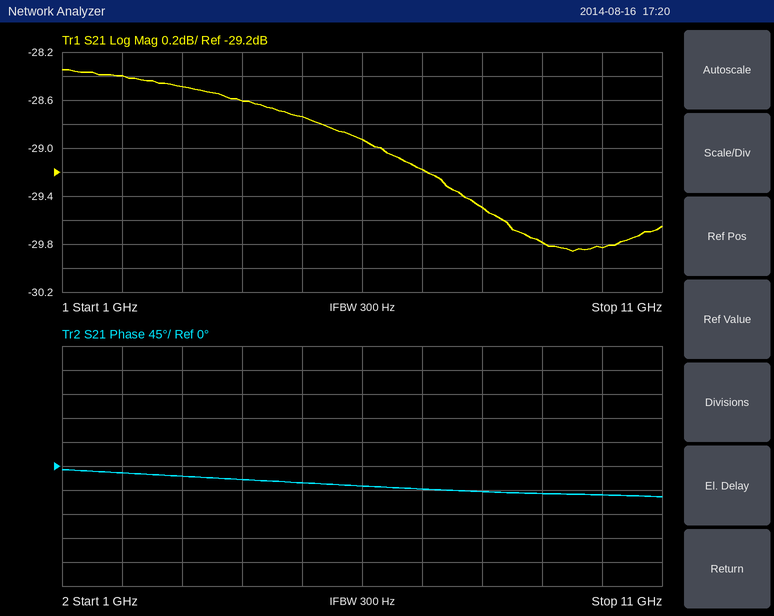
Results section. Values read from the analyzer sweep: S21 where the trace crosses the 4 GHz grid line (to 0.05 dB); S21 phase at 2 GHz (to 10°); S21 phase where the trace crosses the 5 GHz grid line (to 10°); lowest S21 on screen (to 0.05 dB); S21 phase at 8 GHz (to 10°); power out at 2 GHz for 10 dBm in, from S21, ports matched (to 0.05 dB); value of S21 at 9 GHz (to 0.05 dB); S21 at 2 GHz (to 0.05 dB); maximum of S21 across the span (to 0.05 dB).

-28.60 dB
-10°
-30°
-29.85 dB
-50°
-18.40 dBm
-29.80 dB
-28.40 dB
-28.35 dB
